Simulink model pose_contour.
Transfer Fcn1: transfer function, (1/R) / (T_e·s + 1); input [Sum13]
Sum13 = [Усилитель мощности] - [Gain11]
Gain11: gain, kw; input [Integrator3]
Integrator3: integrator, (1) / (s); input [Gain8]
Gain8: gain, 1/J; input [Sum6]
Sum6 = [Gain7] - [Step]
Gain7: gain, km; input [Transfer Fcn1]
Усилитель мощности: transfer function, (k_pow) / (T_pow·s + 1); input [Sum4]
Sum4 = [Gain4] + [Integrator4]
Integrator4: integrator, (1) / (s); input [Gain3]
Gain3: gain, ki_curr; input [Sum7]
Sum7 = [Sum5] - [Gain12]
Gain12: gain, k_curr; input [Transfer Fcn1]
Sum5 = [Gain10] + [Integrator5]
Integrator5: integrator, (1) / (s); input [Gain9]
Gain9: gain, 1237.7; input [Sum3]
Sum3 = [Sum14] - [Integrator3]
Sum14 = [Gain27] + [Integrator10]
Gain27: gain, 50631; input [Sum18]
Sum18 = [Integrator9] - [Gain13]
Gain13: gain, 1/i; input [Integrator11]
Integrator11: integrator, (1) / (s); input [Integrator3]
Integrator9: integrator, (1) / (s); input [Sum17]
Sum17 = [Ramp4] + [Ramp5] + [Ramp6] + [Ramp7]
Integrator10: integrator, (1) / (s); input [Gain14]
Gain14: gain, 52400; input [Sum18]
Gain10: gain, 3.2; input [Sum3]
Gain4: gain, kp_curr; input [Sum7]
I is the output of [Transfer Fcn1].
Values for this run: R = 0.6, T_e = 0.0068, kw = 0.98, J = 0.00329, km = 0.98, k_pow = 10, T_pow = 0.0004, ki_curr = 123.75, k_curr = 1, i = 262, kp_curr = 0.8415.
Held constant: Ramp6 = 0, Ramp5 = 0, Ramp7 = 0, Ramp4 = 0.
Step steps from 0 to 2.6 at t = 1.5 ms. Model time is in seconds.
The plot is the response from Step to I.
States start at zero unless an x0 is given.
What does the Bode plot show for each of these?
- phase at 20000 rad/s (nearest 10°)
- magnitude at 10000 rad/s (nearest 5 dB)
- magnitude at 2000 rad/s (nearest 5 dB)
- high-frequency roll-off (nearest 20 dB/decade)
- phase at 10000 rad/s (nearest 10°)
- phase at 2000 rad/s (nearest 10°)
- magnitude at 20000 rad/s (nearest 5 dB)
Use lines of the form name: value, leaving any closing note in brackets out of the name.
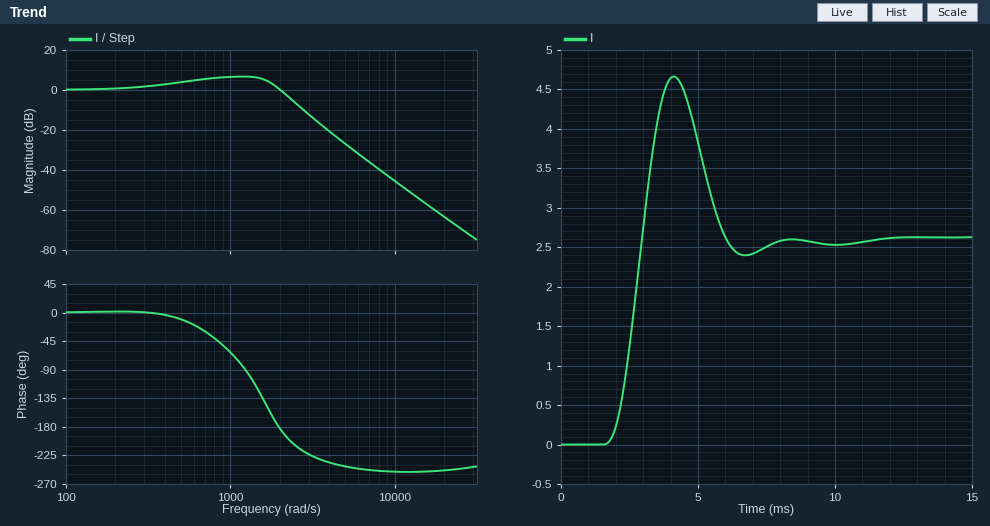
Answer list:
phase at 20000 rad/s: -250°
magnitude at 10000 rad/s: -45 dB
magnitude at 2000 rad/s: 0 dB
high-frequency roll-off: -60 dB/decade
phase at 10000 rad/s: -250°
phase at 2000 rad/s: -180°
magnitude at 20000 rad/s: -65 dB
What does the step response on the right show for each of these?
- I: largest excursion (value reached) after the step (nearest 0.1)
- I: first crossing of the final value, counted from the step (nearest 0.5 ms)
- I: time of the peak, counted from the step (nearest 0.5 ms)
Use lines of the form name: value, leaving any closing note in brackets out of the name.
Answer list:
I: largest excursion (value reached) after the step: 4.7
I: first crossing of the final value, counted from the step: 1.5 ms
I: time of the peak, counted from the step: 2.5 ms
